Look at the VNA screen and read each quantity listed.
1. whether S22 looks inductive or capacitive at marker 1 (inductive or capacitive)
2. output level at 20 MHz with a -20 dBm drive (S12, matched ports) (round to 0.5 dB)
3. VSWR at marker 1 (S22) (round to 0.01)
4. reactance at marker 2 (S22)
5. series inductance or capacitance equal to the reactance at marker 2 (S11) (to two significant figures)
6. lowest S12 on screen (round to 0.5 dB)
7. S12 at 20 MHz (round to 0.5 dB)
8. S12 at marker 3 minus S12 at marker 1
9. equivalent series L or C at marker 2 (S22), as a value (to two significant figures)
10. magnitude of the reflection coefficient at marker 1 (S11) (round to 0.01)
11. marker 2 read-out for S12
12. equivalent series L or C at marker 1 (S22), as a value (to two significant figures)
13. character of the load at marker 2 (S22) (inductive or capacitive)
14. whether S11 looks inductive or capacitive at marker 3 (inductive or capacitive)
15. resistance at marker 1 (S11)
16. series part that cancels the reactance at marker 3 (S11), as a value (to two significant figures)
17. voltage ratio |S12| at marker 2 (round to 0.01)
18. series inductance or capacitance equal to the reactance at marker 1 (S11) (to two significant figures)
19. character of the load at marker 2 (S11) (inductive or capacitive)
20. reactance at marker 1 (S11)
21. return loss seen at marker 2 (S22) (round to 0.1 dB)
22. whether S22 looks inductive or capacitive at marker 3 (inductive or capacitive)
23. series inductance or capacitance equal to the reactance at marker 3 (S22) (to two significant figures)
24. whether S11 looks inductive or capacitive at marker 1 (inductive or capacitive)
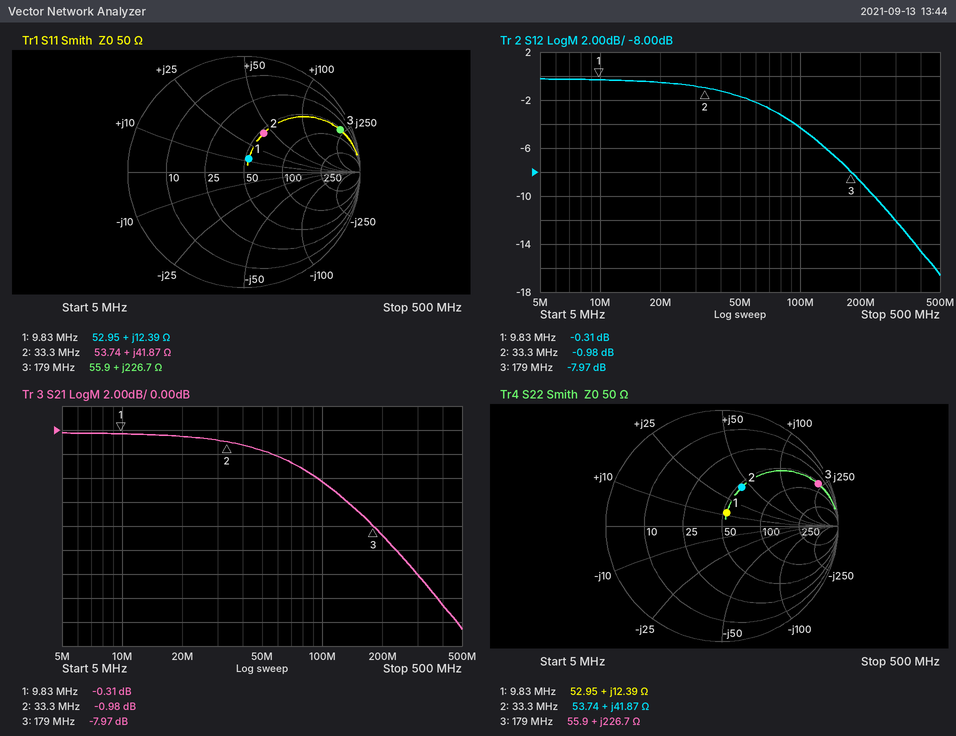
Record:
inductive
-20.5 dBm
1.28
+41.87 Ω
200 nH
-16.5 dB
-0.5 dB
-7.66 dB
200 nH
0.12
-0.98 dB
200 nH
inductive
inductive
52.95 Ω
3.9 pF
0.89
200 nH
inductive
+12.39 Ω
8.5 dB
inductive
200 nH
inductive
